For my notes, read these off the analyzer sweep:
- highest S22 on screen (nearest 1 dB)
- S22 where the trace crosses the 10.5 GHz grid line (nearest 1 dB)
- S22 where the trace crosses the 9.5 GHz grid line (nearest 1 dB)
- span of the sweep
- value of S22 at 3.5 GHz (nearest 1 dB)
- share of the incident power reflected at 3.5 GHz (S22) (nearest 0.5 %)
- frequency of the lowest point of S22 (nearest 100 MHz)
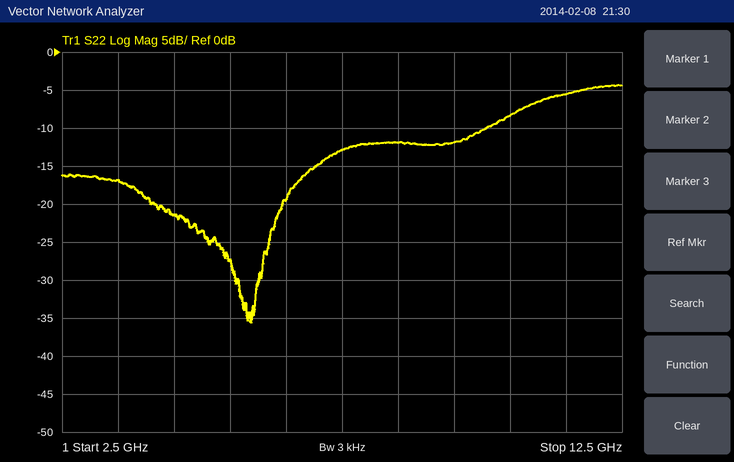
-4 dB
-8 dB
-12 dB
10 GHz
-17 dB
2.0 %
5.9 GHz
